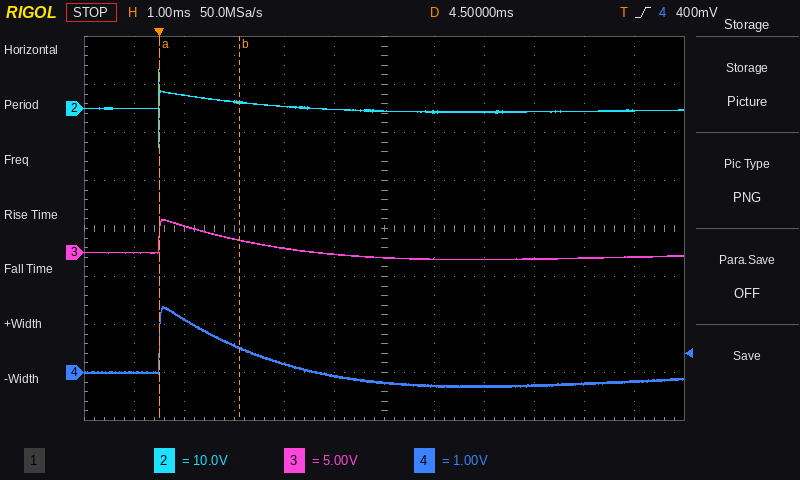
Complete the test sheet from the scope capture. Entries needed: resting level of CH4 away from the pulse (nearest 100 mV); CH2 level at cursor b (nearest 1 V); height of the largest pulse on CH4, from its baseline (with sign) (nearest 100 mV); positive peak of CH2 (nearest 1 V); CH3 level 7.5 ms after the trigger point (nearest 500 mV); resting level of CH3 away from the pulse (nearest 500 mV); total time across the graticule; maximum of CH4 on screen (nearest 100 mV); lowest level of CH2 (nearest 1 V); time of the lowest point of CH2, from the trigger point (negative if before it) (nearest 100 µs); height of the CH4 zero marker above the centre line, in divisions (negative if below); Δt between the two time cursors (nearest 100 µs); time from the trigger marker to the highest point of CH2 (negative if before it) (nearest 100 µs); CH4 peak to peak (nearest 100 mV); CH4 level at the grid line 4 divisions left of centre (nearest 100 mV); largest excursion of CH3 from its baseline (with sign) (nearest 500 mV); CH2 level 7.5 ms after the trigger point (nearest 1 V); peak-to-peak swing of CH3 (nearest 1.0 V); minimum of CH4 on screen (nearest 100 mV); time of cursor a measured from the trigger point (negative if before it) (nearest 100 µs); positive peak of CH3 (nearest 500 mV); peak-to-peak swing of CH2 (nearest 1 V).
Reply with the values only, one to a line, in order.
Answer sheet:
-200 mV
1 V
+1.6 V
8 V
-500 mV
-500 mV
12 ms
1.4 V
-8 V
0.0 ms
-3.0 div
1.6 ms
0.0 ms
1.7 V
1.1 V
+4.0 V
-1 V
4.0 V
-300 mV
0.0 ms
3.5 V
16 V
